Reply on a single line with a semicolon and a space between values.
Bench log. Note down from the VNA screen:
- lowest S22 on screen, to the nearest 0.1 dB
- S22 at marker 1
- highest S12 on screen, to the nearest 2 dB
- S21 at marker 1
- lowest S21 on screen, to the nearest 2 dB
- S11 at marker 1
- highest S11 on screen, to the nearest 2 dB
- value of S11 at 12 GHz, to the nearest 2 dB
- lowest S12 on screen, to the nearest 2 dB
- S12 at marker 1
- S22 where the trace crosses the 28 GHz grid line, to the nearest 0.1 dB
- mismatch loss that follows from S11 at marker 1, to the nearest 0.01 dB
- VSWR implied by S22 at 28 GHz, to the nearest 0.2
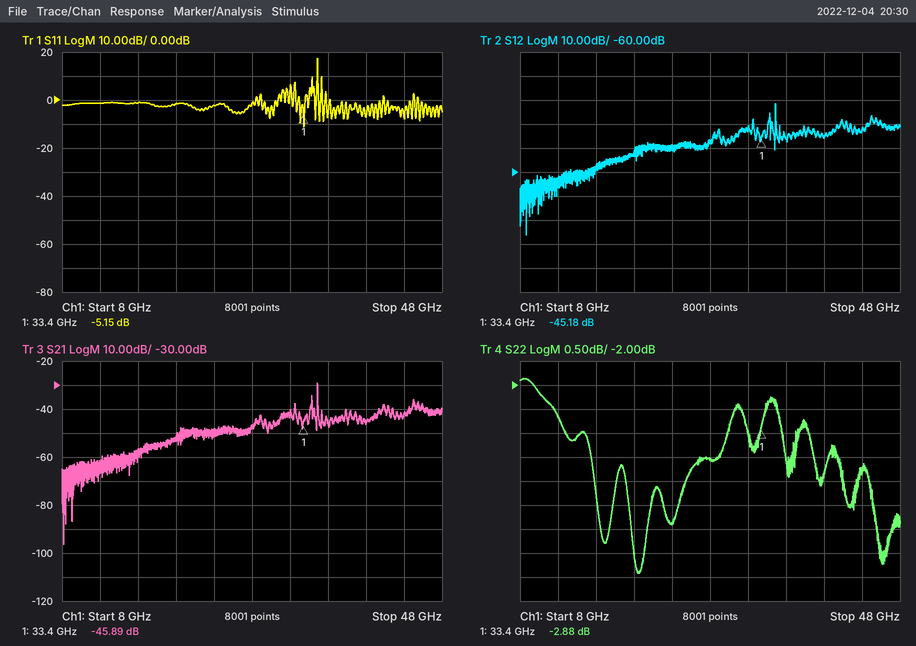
-5.9 dB; -2.88 dB; -32 dB; -45.89 dB; -96 dB; -5.15 dB; 18 dB; -2 dB; -86 dB; -45.18 dB; -3.5 dB; 1.58 dB; 5.0
